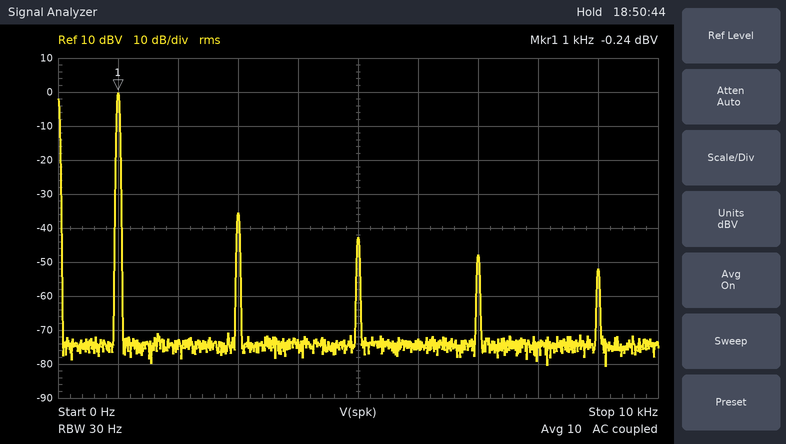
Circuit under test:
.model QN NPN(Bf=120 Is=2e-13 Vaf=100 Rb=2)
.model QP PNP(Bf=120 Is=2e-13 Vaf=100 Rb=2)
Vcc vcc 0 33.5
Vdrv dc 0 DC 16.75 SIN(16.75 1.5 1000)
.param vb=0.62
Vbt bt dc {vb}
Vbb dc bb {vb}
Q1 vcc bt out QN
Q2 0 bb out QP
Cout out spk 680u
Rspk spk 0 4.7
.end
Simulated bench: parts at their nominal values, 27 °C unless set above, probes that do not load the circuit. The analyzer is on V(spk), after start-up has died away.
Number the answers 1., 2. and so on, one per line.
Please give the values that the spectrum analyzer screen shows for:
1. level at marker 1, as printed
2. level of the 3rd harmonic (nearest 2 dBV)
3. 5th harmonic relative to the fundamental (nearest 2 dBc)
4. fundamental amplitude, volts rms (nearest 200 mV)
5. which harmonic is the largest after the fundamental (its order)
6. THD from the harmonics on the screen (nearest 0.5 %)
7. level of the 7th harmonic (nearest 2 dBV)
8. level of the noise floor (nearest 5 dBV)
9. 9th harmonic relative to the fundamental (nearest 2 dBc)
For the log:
1. -0.24 dBV
2. -36 dBV
3. -42 dBc
4. 1.0 V
5. 3
6. 2.0 %
7. -48 dBV
8. -75 dBV
9. -52 dBc
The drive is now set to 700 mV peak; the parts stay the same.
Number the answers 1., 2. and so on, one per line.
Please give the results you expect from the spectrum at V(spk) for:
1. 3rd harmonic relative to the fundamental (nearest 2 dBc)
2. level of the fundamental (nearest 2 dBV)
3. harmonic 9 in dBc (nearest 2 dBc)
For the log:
1. -32 dBc
2. -8 dBV
3. -54 dBc
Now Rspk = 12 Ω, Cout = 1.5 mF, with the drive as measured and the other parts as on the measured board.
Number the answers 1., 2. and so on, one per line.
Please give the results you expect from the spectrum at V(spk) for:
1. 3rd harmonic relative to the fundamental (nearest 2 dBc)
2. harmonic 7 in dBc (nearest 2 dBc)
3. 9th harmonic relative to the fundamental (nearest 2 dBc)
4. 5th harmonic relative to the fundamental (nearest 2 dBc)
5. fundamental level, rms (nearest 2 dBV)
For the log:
1. -40 dBc
2. -54 dBc
3. -60 dBc
4. -48 dBc
5. 0 dBV
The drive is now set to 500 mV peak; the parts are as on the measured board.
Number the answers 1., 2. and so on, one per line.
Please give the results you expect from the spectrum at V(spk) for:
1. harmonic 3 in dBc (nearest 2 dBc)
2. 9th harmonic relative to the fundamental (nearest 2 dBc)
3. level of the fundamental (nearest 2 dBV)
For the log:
1. -32 dBc
2. -56 dBc
3. -10 dBV
